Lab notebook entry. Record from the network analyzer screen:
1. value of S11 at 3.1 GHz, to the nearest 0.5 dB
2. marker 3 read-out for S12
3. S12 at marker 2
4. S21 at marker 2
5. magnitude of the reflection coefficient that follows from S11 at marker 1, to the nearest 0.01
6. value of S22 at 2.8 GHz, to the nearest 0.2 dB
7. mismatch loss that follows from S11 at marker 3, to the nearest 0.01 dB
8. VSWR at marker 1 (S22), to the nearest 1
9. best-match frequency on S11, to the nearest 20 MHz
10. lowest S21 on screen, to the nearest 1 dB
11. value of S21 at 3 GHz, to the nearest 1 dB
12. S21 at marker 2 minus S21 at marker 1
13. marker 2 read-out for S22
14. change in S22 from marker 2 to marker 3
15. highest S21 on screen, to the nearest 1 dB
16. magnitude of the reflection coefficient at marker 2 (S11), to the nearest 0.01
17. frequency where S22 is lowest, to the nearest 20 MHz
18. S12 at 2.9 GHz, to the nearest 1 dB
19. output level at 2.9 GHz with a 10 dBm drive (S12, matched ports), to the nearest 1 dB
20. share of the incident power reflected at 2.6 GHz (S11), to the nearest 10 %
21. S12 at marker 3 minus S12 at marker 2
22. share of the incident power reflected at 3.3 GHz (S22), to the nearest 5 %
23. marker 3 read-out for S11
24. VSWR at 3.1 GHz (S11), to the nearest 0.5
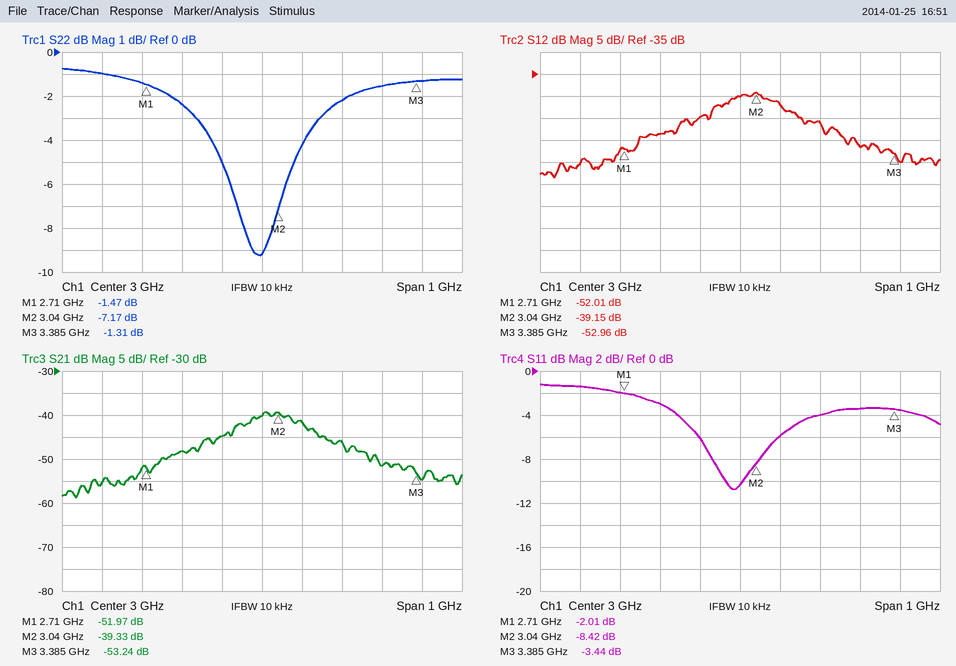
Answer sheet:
-6.0 dB
-52.96 dB
-39.15 dB
-39.33 dB
0.79
-2.4 dB
2.62 dB
12
2.98 GHz
-59 dB
-40 dB
12.64 dB
-7.17 dB
5.86 dB
-39 dB
0.38
3.00 GHz
-45 dB
-35 dBm
70 %
-13.81 dB
70 %
-3.44 dB
3.0
